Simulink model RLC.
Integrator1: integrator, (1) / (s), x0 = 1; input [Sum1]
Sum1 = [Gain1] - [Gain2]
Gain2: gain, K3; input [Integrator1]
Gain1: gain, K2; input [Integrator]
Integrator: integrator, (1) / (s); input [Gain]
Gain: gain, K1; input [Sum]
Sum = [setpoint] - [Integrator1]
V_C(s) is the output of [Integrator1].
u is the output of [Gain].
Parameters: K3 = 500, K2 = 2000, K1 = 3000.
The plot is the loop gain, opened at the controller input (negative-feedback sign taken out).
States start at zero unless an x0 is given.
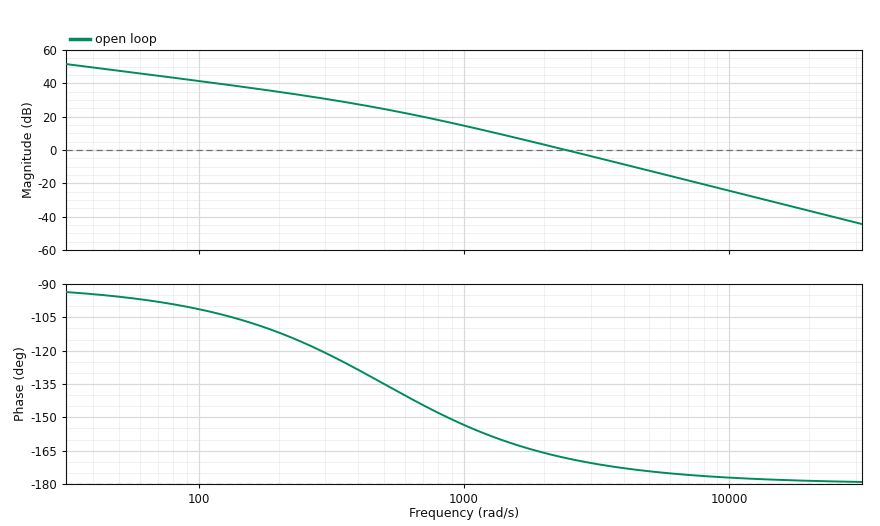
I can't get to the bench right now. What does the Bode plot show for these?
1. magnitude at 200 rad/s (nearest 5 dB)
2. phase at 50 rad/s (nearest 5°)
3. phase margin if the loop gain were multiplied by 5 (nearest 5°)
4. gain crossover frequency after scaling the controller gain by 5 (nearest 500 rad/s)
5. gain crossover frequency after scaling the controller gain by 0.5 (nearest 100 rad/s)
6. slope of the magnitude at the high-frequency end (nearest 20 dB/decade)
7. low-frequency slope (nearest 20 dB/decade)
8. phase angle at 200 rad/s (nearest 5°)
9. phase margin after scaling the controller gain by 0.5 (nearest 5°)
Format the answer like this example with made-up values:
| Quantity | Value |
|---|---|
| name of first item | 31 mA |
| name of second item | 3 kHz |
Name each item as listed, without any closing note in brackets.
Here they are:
| Quantity | Value |
|---|---|
| magnitude at 200 rad/s | 35 dB |
| phase at 50 rad/s | -95° |
| phase margin if the loop gain were multiplied by 5 | 5° |
| gain crossover frequency after scaling the controller gain by 5 | 5500 rad/s |
| gain crossover frequency after scaling the controller gain by 0.5 | 1700 rad/s |
| slope of the magnitude at the high-frequency end | -40 dB/decade |
| low-frequency slope | -20 dB/decade |
| phase angle at 200 rad/s | -110° |
| phase margin after scaling the controller gain by 0.5 | 15° |
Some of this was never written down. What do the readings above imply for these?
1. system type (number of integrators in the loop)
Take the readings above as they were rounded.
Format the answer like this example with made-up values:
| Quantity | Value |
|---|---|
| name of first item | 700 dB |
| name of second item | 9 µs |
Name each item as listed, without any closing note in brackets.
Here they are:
| Quantity | Value |
|---|---|
| system type | 1 |
